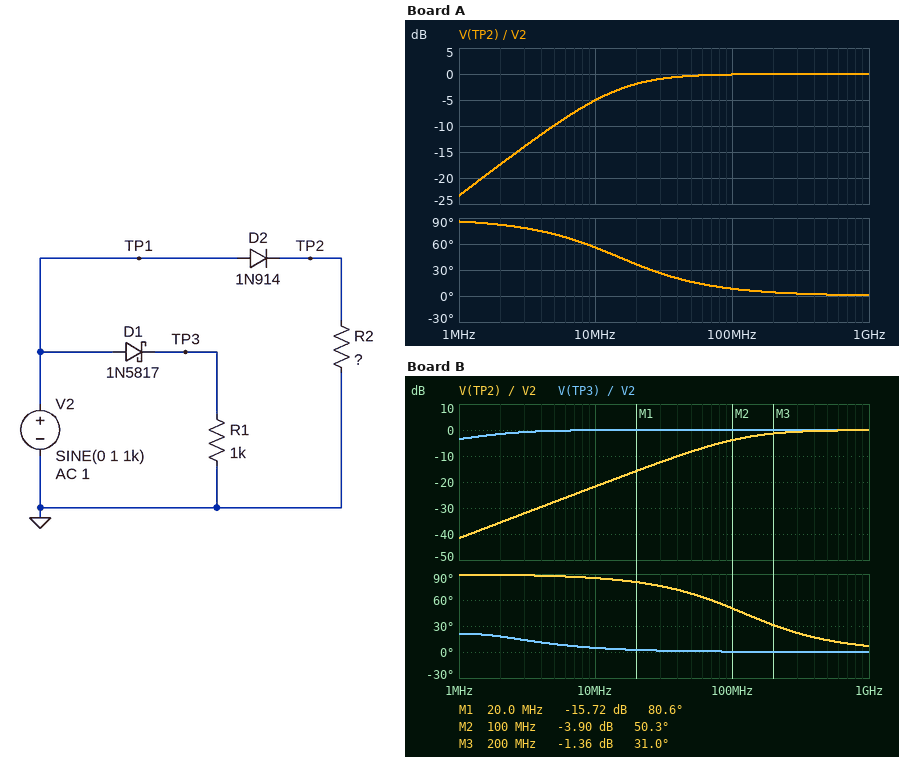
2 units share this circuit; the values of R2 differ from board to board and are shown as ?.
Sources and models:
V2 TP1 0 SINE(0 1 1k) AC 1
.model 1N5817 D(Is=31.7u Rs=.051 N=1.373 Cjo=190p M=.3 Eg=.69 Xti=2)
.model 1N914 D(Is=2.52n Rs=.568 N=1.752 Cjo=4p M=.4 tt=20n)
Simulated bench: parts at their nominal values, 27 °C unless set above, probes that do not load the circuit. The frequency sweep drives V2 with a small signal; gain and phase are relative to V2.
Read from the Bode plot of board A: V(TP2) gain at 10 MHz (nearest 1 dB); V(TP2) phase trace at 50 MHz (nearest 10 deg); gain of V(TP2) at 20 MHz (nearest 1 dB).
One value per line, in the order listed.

-5 dB
20 deg
-2 dB
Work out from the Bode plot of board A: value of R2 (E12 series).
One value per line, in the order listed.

2.7 kΩ
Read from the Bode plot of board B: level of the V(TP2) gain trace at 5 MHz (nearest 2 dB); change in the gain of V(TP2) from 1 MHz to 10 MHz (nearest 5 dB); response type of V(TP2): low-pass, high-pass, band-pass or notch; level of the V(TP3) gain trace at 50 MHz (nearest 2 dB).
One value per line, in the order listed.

-28 dB
20 dB
high-pass
0 dB
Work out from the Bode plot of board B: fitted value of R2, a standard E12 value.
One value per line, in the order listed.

330 Ω
